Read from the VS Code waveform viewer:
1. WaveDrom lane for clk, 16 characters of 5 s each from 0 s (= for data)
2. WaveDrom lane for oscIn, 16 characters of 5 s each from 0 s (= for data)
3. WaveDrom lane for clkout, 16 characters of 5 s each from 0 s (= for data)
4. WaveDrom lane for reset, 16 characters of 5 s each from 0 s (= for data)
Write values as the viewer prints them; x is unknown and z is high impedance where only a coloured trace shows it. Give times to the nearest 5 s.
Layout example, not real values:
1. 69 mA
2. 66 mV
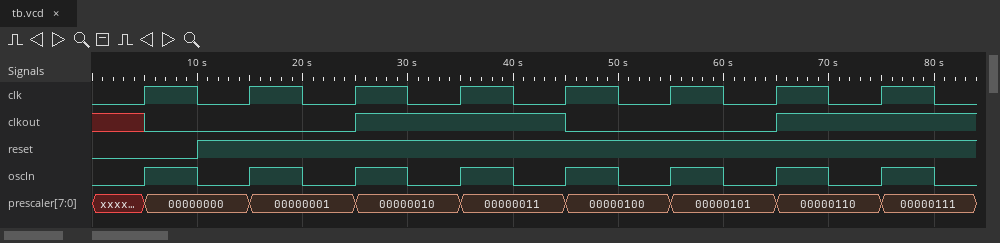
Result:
1. {name: 'clk', wave: '0101010101010101'}
2. {name: 'oscIn', wave: '0101010101010101'}
3. {name: 'clkout', wave: 'x0...1...0...1..'}
4. {name: 'reset', wave: '0.1.............'}
